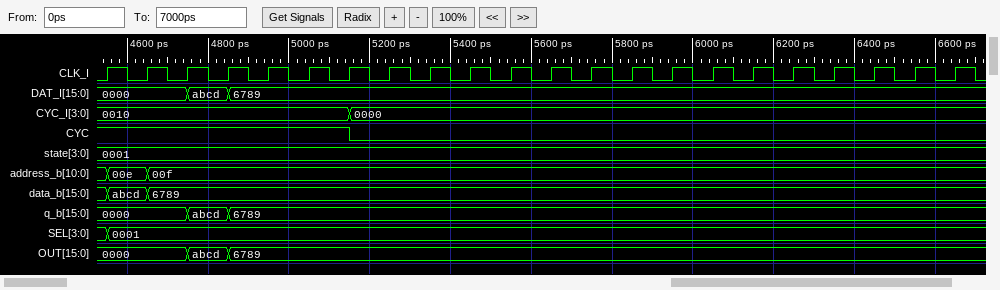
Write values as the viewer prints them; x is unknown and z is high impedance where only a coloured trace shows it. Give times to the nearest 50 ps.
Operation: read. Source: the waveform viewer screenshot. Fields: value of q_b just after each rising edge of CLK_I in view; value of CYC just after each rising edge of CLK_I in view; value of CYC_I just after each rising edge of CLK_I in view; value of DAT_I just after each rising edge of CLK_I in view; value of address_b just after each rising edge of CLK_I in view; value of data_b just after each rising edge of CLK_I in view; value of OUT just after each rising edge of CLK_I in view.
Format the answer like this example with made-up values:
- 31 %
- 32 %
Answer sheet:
- 0000, 0000, abcd, 6789, 6789, 6789, 6789, 6789, 6789, 6789, 6789, 6789, 6789, 6789, 6789, 6789, 6789, 6789, 6789, 6789, 6789, 6789
- 1 1 1 1 1 1 0 0 0 0 0 0 0 0 0 0 0 0 0 0 0 0
- 0010, 0010, 0010, 0010, 0010, 0010, 0000, 0000, 0000, 0000, 0000, 0000, 0000, 0000, 0000, 0000, 0000, 0000, 0000, 0000, 0000, 0000
- 0000, 0000, abcd, 6789, 6789, 6789, 6789, 6789, 6789, 6789, 6789, 6789, 6789, 6789, 6789, 6789, 6789, 6789, 6789, 6789, 6789, 6789
- 00e, 00f, 00f, 00f, 00f, 00f, 00f, 00f, 00f, 00f, 00f, 00f, 00f, 00f, 00f, 00f, 00f, 00f, 00f, 00f, 00f, 00f
- abcd, 6789, 6789, 6789, 6789, 6789, 6789, 6789, 6789, 6789, 6789, 6789, 6789, 6789, 6789, 6789, 6789, 6789, 6789, 6789, 6789, 6789
- 0000, 0000, abcd, 6789, 6789, 6789, 6789, 6789, 6789, 6789, 6789, 6789, 6789, 6789, 6789, 6789, 6789, 6789, 6789, 6789, 6789, 6789
